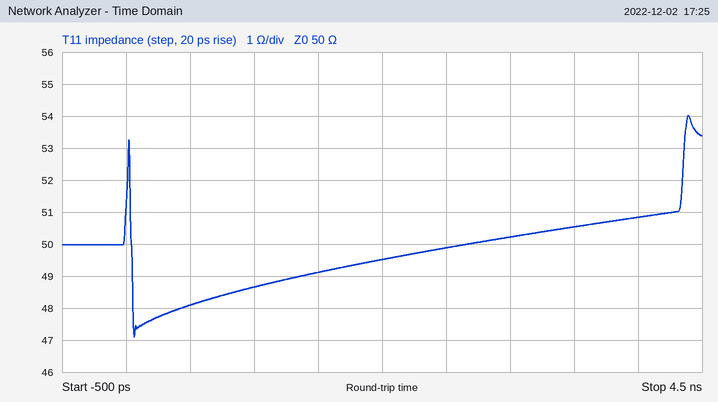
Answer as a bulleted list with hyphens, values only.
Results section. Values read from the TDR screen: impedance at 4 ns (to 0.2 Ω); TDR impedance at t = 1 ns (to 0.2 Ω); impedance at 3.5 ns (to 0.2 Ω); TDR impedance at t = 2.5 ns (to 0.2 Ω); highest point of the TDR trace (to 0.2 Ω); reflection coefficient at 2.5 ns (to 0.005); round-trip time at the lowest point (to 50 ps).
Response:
- 50.8 Ω
- 48.6 Ω
- 50.6 Ω
- 49.8 Ω
- 54.0 Ω
- 0.000
- 50 ps
